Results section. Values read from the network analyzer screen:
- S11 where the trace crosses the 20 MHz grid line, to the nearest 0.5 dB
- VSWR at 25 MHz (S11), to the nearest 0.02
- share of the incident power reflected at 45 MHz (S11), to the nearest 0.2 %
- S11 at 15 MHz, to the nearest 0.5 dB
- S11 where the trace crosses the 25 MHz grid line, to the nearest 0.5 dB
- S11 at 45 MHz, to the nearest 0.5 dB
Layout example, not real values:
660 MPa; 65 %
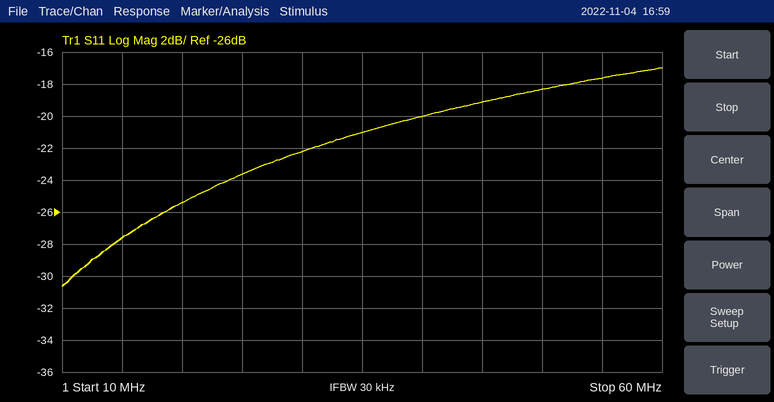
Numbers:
-25.5 dB; 1.14; 1.2 %; -27.5 dB; -23.5 dB; -19.0 dB
